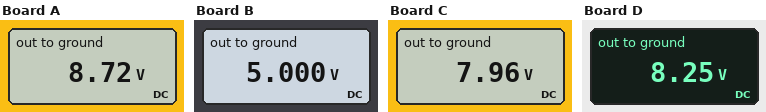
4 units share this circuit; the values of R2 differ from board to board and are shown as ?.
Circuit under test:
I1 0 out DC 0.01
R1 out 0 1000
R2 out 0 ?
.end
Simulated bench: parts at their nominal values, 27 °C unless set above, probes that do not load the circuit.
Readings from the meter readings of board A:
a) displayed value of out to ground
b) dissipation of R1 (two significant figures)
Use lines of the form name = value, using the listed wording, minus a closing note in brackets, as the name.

displayed value of out to ground = 8.72 V
dissipation of R1 = 76 mW
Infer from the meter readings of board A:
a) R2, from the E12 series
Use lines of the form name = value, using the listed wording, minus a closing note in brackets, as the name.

R2, from the E12 series = 6.8 kΩ
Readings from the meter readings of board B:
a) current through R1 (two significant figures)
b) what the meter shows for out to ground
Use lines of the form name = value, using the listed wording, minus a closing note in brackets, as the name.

current through R1 = 5.0 mA
what the meter shows for out to ground = 5.000 V
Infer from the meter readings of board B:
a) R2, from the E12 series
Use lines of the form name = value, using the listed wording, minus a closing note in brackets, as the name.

R2, from the E12 series = 1 kΩ
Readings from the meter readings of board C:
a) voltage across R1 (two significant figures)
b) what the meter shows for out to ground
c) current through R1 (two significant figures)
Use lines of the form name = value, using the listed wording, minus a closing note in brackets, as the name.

voltage across R1 = 8.0 V
what the meter shows for out to ground = 7.96 V
current through R1 = 8.0 mA
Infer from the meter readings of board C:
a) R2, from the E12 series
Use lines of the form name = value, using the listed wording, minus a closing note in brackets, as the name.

R2, from the E12 series = 3.9 kΩ
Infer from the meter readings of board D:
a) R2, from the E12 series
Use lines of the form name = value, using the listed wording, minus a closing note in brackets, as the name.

R2, from the E12 series = 4.7 kΩ
